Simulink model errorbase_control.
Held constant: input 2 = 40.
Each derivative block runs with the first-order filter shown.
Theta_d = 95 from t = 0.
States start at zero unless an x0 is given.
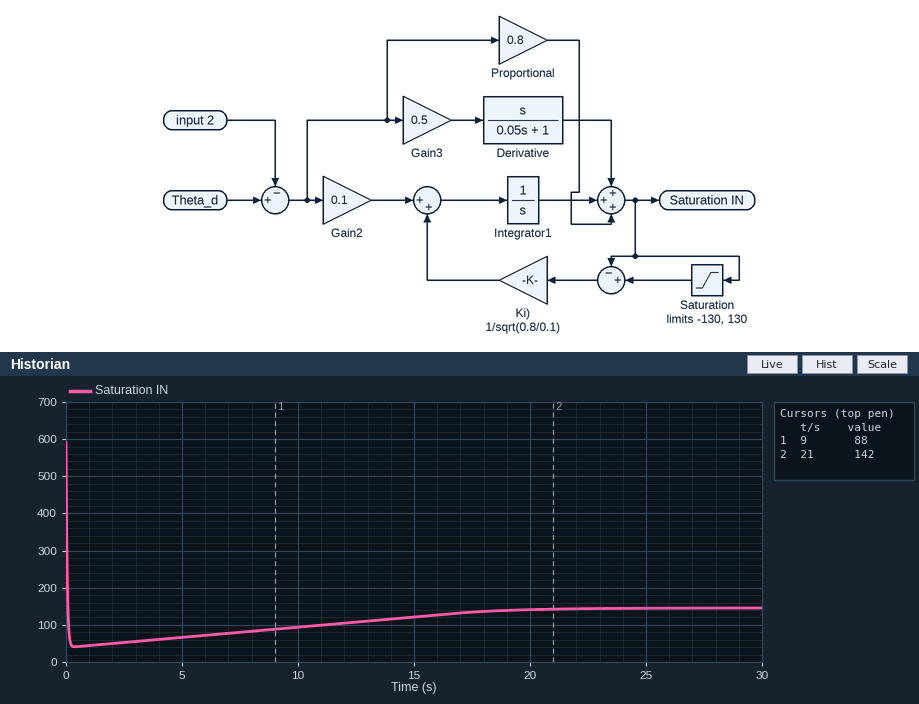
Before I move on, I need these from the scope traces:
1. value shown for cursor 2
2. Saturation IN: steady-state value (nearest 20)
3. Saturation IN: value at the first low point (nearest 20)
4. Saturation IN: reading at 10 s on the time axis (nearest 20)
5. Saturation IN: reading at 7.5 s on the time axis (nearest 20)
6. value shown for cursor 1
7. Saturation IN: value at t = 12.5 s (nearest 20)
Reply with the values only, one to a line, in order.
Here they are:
142
140
40
100
80
88
100
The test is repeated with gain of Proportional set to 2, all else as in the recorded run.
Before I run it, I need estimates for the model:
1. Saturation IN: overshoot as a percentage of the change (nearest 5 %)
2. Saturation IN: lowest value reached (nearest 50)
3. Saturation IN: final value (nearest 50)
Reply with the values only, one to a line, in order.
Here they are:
10 %
100
150
